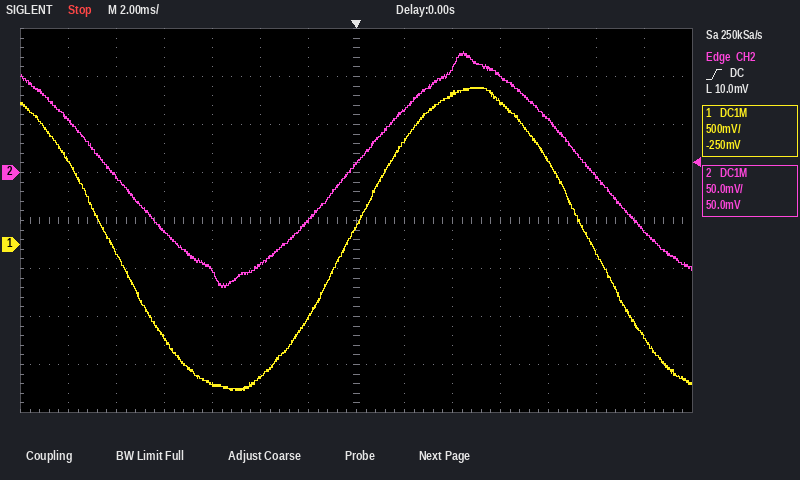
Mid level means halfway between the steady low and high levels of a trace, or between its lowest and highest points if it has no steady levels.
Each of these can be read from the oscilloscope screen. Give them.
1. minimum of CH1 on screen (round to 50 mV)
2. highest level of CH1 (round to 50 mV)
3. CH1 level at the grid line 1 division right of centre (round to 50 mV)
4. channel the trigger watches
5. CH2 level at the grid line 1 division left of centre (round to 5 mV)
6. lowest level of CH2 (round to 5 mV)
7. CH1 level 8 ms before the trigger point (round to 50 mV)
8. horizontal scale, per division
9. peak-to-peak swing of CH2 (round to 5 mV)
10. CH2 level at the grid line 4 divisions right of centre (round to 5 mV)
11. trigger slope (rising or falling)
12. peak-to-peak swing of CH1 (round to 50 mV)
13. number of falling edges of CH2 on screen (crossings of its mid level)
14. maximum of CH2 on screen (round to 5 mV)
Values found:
-1.50 V
1.65 V
1.10 V
CH2
-50 mV
-120 mV
-950 mV
2 ms
245 mV
55 mV
rising
3.15 V
2
125 mV
